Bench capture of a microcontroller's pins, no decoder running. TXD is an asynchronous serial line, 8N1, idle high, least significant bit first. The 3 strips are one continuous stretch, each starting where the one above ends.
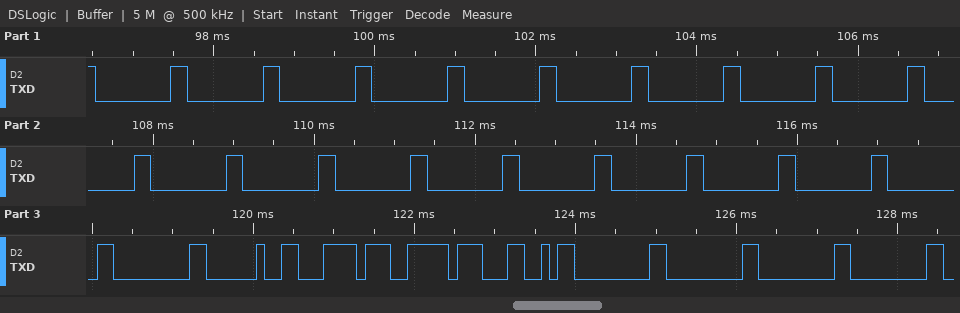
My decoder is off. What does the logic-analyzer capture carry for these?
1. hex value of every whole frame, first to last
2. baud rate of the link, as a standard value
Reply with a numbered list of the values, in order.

1. 00 00 00 00 00 00 00 00 00 00 00 00 00 00 00 00 00 00 00 00 20 BC BE 4C 00 00 00 00
2. 9600 baud
